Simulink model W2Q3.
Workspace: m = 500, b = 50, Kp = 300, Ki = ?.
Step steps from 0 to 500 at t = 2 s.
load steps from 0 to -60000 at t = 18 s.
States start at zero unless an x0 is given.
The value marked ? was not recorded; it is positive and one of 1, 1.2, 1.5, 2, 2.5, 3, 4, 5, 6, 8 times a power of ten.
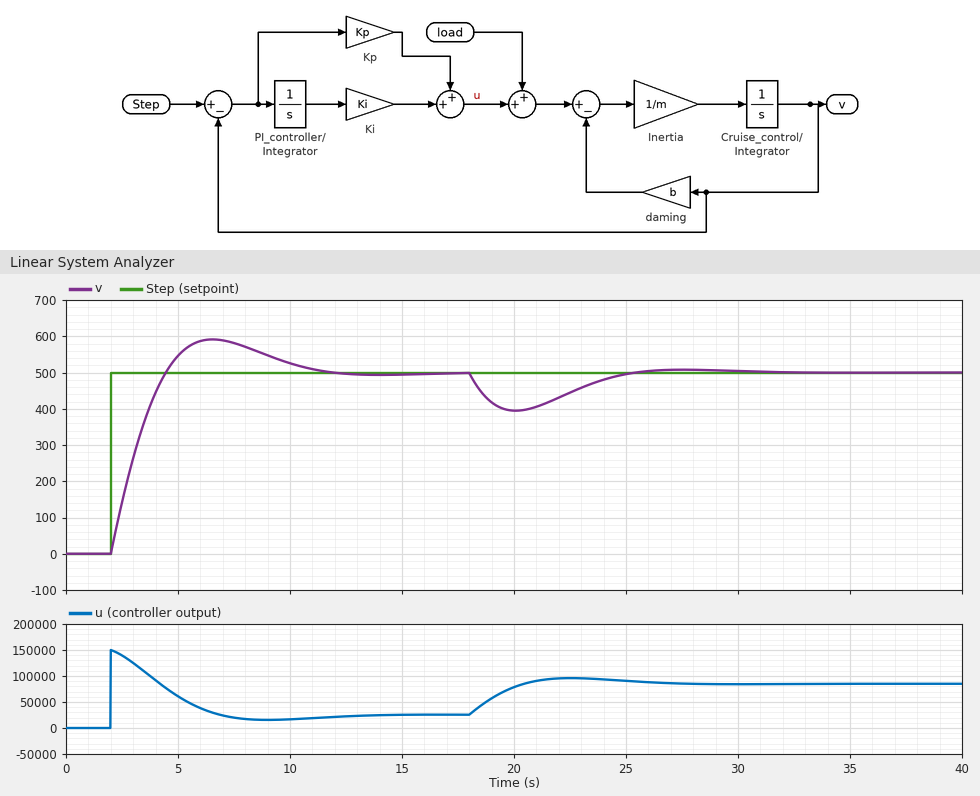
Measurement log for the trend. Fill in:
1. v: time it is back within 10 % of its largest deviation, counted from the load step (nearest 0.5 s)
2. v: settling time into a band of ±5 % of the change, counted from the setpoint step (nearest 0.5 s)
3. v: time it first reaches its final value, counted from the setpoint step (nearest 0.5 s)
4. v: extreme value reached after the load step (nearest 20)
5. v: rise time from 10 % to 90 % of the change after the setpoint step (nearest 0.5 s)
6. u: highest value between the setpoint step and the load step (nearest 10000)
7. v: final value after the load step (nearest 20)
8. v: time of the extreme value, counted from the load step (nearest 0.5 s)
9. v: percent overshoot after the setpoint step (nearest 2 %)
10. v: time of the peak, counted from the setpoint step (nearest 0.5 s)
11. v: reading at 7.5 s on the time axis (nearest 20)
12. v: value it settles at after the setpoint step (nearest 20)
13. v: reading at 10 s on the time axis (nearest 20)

6.5 s
8.0 s
2.5 s
400
2.0 s
150000
500
2.0 s
18 %
4.5 s
580
500
520
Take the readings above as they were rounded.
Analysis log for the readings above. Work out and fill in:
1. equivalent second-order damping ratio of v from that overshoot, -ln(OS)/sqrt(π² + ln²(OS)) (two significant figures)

0.48
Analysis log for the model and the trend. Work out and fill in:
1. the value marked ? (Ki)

150
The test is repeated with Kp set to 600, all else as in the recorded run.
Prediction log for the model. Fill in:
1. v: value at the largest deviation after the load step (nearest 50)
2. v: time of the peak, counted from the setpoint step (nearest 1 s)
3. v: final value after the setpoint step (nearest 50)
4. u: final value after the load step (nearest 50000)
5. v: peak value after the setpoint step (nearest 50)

450
4 s
500
100000
550
